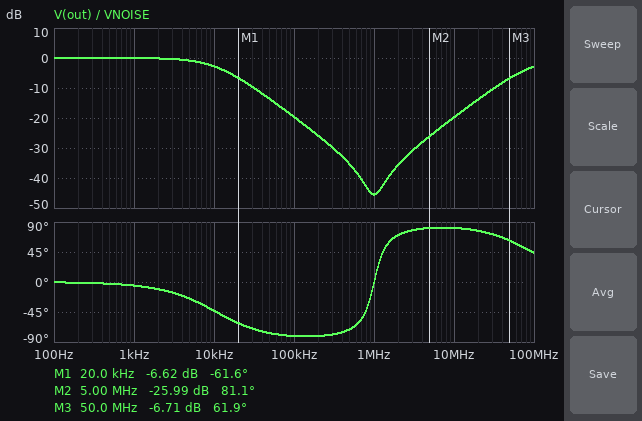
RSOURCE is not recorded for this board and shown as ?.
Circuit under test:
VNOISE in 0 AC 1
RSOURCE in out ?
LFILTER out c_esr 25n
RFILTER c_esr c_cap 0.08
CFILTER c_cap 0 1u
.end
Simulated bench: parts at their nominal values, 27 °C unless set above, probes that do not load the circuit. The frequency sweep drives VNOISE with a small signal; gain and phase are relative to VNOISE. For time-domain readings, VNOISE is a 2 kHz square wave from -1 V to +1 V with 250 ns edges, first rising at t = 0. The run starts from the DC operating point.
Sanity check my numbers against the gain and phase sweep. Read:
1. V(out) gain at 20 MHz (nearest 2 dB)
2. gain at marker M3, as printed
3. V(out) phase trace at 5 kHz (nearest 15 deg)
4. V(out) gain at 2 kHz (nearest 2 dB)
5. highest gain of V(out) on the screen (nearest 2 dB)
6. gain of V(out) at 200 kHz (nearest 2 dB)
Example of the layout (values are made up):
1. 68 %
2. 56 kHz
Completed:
1. -14 dB
2. -6.71 dB
3. -30 deg
4. 0 dB
5. 0 dB
6. -26 dB
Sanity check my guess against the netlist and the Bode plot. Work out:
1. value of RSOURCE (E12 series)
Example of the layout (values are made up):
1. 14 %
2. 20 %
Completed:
1. 15 Ω
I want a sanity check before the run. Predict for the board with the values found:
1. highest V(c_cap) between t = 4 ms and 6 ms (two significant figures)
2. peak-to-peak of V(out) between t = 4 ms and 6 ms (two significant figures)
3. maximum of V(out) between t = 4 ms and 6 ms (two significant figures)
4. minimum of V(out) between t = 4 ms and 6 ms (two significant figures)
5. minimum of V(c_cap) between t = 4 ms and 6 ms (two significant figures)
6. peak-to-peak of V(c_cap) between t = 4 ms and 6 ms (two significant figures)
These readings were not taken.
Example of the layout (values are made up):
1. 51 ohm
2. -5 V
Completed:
1. 1.0 V
2. 2.0 V
3. 1.0 V
4. -1.0 V
5. -1.0 V
6. 2.0 V
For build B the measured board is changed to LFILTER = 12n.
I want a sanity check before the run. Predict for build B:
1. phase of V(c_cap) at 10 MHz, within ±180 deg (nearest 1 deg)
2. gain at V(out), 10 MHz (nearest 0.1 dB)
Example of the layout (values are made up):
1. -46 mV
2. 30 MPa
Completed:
1. -93 deg
2. -26.2 dB
